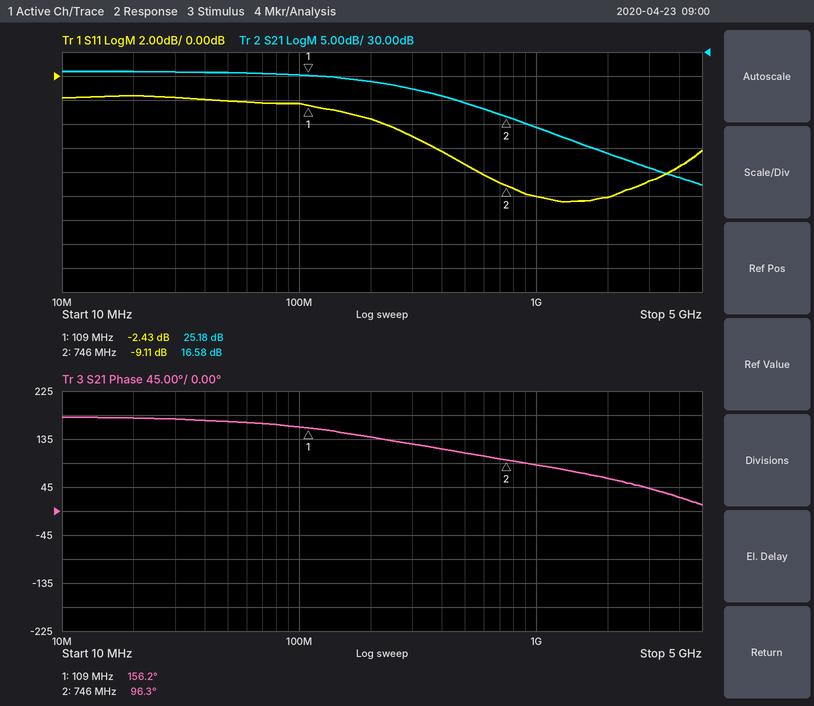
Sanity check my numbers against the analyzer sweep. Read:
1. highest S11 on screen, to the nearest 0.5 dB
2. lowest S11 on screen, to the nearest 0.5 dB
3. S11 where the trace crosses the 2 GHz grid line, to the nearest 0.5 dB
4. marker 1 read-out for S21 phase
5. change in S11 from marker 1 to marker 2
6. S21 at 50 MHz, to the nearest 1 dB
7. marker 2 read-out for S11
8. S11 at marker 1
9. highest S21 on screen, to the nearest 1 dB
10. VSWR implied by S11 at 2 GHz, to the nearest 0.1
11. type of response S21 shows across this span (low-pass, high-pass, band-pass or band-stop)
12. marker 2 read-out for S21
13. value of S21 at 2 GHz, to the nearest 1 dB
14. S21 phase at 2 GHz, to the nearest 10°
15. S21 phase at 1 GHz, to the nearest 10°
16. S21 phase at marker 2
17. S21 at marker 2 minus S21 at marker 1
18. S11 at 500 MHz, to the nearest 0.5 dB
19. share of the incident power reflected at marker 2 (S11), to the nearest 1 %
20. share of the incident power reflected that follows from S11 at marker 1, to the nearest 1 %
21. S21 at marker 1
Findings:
-1.5 dB
-10.5 dB
-10.0 dB
156.2°
-6.68 dB
26 dB
-9.11 dB
-2.43 dB
26 dB
1.9
low-pass
16.58 dB
9 dB
60°
90°
96.3°
-8.60 dB
-7.5 dB
12 %
57 %
25.18 dB
